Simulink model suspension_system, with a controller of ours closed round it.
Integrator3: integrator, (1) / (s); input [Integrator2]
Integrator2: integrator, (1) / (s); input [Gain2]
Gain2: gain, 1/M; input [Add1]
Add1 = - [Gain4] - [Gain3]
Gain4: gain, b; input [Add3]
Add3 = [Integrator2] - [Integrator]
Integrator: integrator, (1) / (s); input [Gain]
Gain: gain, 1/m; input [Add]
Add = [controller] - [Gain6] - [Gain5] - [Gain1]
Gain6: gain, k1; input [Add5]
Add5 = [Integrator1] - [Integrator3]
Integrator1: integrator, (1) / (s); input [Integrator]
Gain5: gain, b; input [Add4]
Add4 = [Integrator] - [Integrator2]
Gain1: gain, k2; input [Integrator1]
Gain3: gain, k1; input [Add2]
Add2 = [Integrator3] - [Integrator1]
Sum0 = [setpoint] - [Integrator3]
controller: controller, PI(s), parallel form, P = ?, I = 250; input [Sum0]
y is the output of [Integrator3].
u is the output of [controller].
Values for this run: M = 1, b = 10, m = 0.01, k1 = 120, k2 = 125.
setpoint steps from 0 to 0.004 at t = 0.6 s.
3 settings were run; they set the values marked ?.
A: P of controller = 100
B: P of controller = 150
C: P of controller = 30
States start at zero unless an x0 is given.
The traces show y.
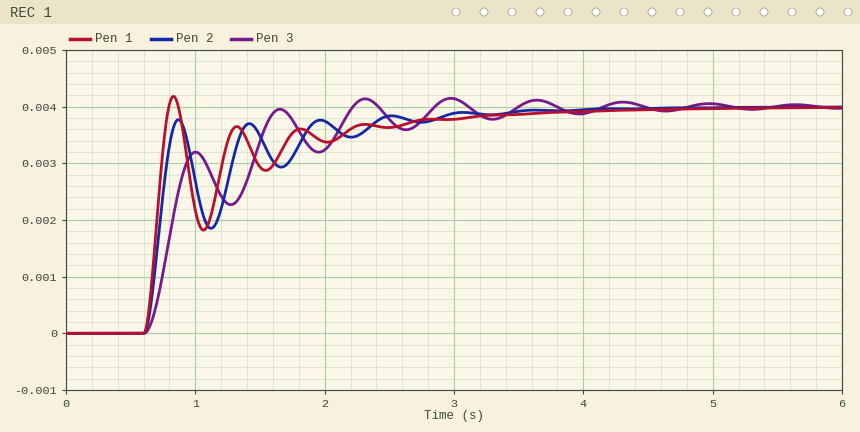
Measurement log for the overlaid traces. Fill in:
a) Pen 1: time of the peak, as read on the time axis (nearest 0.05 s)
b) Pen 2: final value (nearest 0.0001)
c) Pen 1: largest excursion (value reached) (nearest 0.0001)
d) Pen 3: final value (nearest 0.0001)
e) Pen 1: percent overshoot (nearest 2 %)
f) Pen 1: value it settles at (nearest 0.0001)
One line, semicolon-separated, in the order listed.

0.85 s; 0.0040; 0.0042; 0.0040; 4 %; 0.0040
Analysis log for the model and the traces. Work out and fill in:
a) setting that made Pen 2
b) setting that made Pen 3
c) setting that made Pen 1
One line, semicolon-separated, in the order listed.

A; C; B
